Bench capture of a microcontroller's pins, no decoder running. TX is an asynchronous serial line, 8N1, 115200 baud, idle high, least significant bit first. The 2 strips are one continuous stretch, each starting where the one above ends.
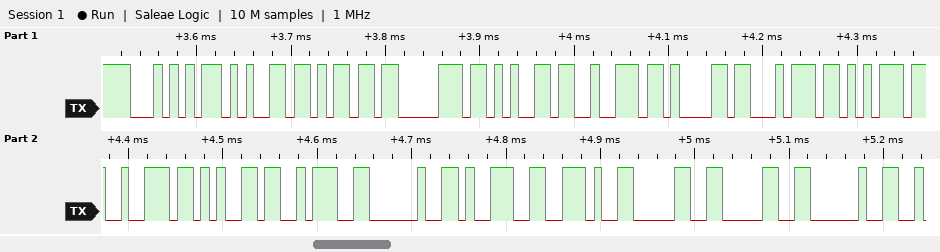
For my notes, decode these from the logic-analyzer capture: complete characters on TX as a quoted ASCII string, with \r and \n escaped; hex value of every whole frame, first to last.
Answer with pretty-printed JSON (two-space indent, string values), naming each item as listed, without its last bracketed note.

{
  "complete characters on TX as a quoted ASCII string, with \\r and \\n escaped": "\"Temperature: 9.00 \"",
  "hex value of every whole frame, first to last": "54 65 6D 70 65 72 61 74 75 72 65 3A 20 39 2E 30 30 20"
}
